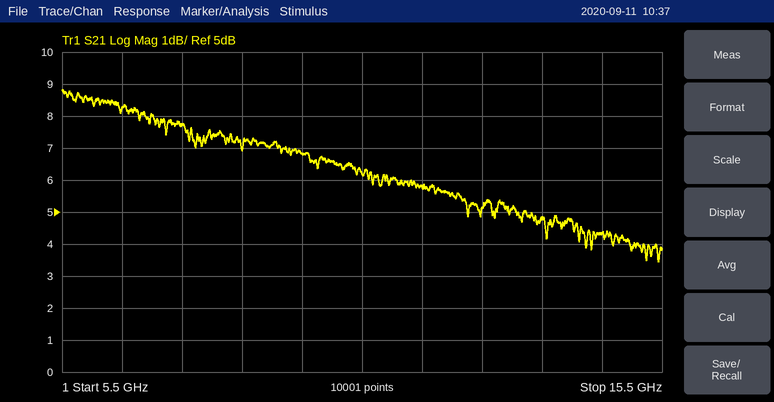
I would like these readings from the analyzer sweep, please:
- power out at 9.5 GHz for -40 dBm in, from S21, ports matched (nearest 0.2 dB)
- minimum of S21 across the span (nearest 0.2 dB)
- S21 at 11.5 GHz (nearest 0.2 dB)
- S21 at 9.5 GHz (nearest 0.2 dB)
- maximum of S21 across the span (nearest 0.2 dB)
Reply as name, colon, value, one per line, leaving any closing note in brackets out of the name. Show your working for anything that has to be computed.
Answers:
power out at 9.5 GHz for -40 dBm in, from S21, ports matched: -40 dBm + (6.8 dB) = -33.2 dBm
minimum of S21 across the span: 3.4 dB
S21 at 11.5 GHz: 5.8 dB
S21 at 9.5 GHz: 6.8 dB
maximum of S21 across the span: 8.8 dB
